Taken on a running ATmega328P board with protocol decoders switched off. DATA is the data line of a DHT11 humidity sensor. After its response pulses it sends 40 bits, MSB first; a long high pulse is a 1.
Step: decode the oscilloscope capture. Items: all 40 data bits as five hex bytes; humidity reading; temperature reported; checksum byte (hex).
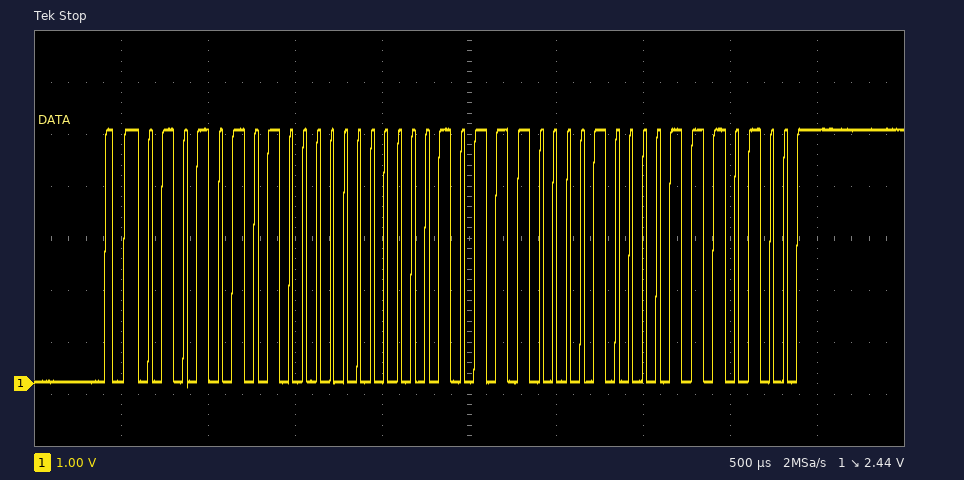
55 00 17 08 74
85 %
23.8 °C
0x74
